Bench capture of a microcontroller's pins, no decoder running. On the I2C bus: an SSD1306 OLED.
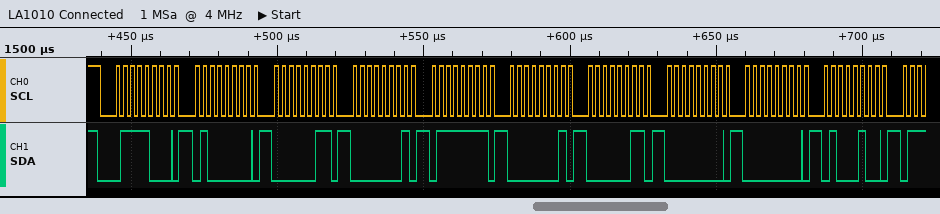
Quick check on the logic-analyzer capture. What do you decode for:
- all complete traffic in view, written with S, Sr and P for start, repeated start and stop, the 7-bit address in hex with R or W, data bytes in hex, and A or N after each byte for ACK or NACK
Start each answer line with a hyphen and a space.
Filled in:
- S 3CW A 40 A 03 A 01 A 7F A 01 A 03 A 00 A 00 A 44 A
